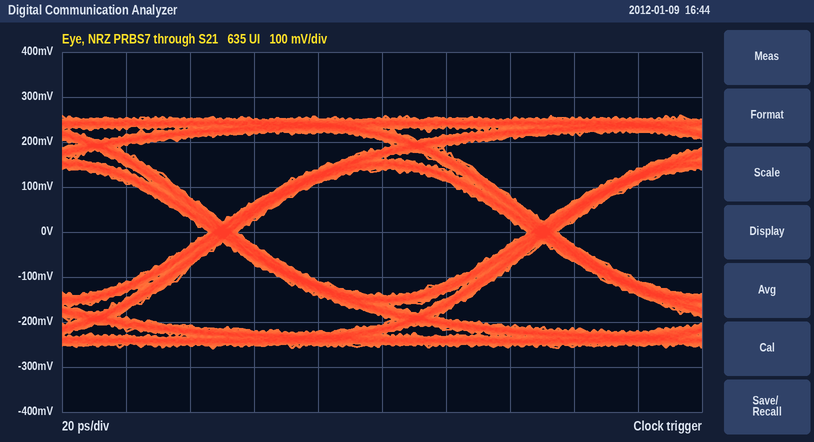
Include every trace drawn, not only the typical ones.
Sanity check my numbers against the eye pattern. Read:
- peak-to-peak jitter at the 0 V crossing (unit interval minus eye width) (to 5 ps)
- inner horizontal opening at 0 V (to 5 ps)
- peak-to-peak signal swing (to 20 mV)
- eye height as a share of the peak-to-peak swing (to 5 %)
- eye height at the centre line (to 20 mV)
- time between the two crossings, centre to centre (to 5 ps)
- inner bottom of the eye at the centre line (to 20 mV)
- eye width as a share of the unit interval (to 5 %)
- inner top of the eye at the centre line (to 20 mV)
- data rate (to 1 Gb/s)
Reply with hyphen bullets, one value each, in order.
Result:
- 10 ps
- 90 ps
- 520 mV
- 55 %
- 280 mV
- 100 ps
- -140 mV
- 90 %
- 140 mV
- 10 Gb/s
